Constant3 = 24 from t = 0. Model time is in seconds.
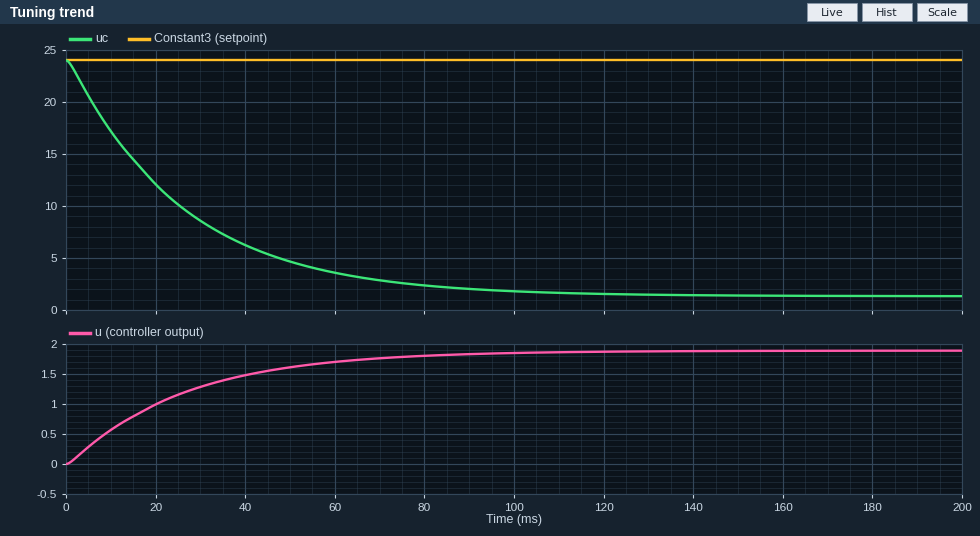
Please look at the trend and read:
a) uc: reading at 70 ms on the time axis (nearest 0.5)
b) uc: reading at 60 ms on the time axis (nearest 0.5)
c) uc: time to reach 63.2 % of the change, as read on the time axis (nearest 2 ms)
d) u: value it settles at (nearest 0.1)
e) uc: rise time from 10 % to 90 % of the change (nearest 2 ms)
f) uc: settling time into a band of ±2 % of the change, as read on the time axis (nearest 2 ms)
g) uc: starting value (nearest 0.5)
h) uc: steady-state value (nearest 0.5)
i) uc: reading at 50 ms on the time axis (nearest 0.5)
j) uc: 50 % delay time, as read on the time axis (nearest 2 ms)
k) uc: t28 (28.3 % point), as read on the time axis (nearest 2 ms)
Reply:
3.0
3.5
26 ms
1.9
56 ms
102 ms
24.0
1.5
4.5
18 ms
10 ms
